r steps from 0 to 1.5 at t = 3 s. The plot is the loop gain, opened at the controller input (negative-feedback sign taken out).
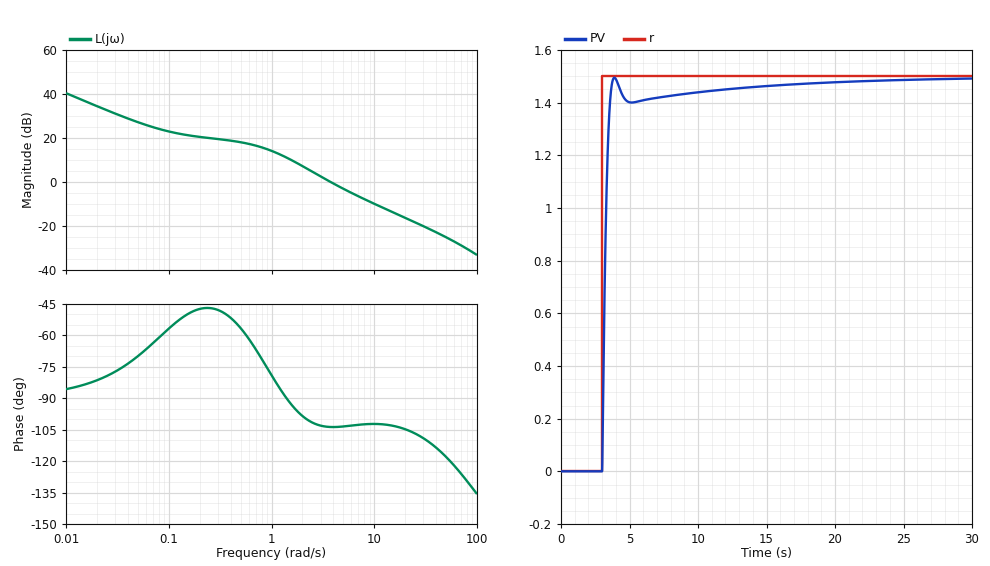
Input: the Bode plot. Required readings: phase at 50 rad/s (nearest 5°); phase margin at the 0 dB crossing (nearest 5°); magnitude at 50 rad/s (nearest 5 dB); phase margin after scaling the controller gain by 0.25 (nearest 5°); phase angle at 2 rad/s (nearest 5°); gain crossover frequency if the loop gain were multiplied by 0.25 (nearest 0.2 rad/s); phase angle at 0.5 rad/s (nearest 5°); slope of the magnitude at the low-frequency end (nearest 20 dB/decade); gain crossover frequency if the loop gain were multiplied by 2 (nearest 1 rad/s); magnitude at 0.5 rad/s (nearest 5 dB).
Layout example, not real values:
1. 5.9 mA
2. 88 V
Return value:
1. -120°
2. 75°
3. -25 dB
4. 95°
5. -100°
6. 1.2 rad/s
7. -55°
8. -20 dB/decade
9. 7 rad/s
10. 20 dB
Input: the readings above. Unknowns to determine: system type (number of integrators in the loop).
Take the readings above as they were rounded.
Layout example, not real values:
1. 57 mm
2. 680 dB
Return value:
1. 1
